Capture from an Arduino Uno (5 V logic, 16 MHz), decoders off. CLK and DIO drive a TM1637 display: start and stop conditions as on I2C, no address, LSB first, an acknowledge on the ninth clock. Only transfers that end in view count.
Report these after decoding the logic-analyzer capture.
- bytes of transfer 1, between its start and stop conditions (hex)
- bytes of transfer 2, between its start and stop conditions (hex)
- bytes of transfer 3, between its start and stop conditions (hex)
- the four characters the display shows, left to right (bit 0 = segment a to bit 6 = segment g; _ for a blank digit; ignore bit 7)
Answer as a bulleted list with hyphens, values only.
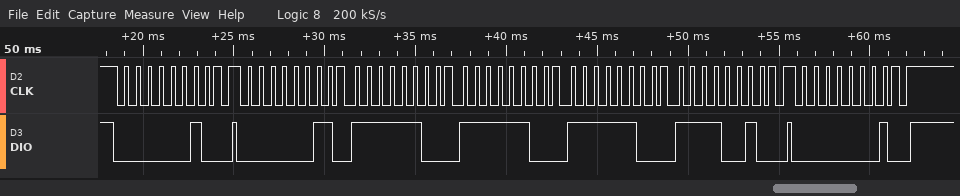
- 40
- C0 3F 3F 3F 4F
- 80
- 0003
